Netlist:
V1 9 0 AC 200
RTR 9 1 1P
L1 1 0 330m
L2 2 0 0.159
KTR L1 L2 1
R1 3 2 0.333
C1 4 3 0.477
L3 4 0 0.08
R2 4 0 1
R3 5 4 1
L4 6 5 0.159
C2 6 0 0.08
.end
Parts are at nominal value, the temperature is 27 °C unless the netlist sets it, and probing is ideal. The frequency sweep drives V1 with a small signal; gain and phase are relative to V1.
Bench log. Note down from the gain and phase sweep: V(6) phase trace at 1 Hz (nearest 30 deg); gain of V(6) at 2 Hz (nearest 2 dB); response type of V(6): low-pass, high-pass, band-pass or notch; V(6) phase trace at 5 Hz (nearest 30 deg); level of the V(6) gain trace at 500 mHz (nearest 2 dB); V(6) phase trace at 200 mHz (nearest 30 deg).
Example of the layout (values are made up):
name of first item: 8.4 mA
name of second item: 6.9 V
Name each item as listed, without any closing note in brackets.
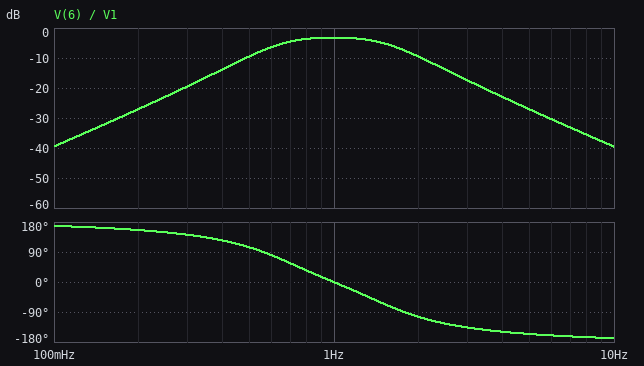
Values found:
V(6) phase trace at 1 Hz: 0 deg
gain of V(6) at 2 Hz: -10 dB
response type of V(6): low-pass, high-pass, band-pass or notch: band-pass
V(6) phase trace at 5 Hz: -150 deg
level of the V(6) gain trace at 500 mHz: -10 dB
V(6) phase trace at 200 mHz: 150 deg
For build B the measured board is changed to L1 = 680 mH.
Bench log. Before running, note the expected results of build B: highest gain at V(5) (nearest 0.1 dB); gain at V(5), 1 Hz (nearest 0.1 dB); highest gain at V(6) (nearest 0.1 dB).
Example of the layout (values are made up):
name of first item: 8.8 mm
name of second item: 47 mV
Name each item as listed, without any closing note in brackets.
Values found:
highest gain at V(5): -8.8 dB
gain at V(5), 1 Hz: -12.4 dB
highest gain at V(6): -6.3 dB
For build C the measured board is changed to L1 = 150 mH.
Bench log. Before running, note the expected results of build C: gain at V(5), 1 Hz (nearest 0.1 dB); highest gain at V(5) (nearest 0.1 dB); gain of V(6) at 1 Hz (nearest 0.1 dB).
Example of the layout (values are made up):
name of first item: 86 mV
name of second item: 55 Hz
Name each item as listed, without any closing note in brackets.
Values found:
gain at V(5), 1 Hz: -5.8 dB
highest gain at V(5): -2.2 dB
gain of V(6) at 1 Hz: 0.2 dB
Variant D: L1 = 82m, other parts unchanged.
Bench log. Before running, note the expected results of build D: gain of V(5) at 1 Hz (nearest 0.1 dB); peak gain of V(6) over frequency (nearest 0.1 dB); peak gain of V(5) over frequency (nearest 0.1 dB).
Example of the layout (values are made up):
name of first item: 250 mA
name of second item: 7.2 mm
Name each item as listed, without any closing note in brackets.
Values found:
gain of V(5) at 1 Hz: -3.2 dB
peak gain of V(6) over frequency: 2.9 dB
peak gain of V(5) over frequency: 0.4 dB
